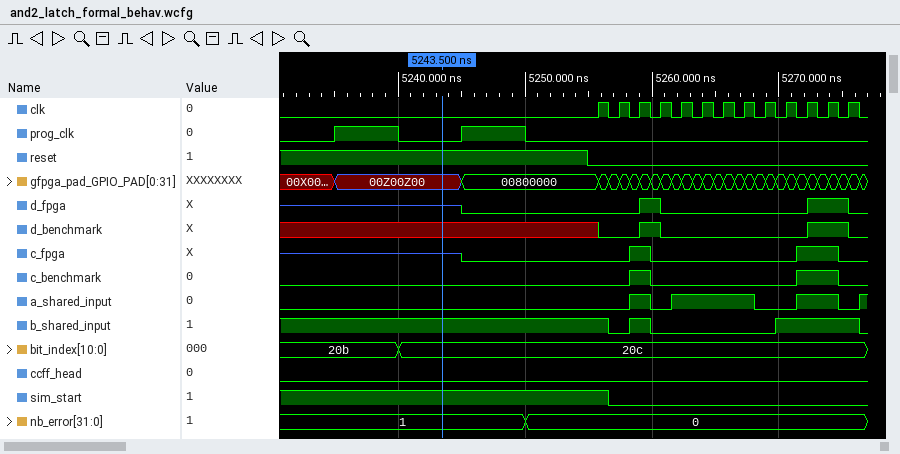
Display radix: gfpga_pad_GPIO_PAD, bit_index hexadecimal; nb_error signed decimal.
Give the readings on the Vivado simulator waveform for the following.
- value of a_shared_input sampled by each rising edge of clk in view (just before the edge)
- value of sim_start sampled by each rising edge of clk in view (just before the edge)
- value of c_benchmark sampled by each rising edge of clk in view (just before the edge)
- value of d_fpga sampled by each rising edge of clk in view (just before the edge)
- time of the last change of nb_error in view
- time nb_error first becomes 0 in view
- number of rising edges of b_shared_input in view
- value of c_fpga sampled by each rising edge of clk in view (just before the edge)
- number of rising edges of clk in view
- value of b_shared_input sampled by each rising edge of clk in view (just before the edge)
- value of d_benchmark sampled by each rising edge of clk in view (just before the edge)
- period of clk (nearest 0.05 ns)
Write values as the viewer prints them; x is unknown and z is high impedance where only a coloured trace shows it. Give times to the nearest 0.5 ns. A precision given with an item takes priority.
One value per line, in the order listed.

0 0 1 0 1 1 1 1 0 0 1 1 0
1 0 0 0 0 0 0 0 0 0 0 0 0
0 0 1 0 0 0 0 0 0 0 1 1 0
0 0 0 1 0 0 0 0 0 0 0 1 1
5250 ns
5250 ns
2
0 0 1 0 0 0 0 0 0 0 1 1 0
13
1 0 1 0 0 0 0 0 0 1 1 1 1
x 0 0 1 0 0 0 0 0 0 0 1 1
1.65 ns
